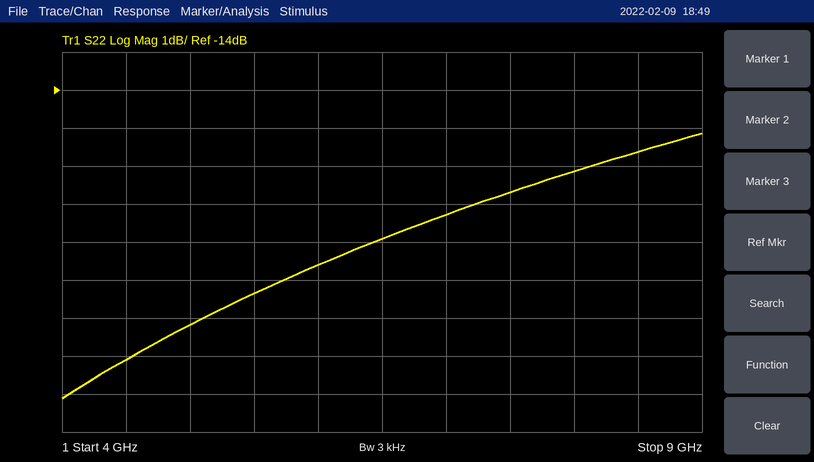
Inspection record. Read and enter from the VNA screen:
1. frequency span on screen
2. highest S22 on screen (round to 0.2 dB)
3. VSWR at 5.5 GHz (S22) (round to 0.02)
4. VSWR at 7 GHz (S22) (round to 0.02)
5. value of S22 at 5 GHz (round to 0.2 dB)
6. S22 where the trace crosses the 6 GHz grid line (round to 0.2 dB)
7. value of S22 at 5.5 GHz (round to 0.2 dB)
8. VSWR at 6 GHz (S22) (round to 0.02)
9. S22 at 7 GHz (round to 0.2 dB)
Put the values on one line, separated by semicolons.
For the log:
5 GHz; -15.2 dB; 1.24; 1.32; -20.2 dB; -18.6 dB; -19.4 dB; 1.26; -17.2 dB
